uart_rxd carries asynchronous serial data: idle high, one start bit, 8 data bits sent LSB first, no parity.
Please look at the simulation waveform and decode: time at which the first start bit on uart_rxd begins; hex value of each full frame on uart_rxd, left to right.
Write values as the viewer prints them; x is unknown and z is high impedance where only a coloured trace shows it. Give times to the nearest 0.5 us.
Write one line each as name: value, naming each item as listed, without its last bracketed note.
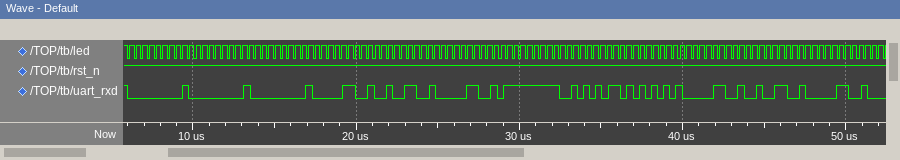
time at which the first start bit on uart_rxd begins: 6 us
hex value of each full frame on uart_rxd, left to right: 00, 00, 00, 30, 32, 30, FF, AA, 55, 30, 32, 30
